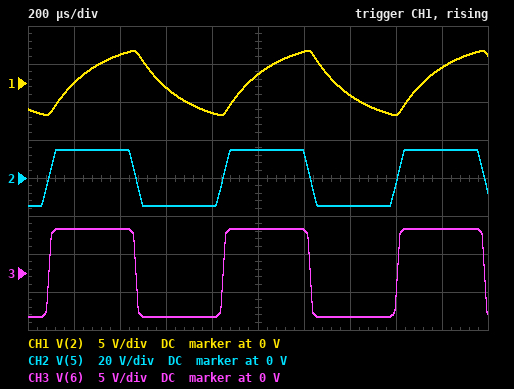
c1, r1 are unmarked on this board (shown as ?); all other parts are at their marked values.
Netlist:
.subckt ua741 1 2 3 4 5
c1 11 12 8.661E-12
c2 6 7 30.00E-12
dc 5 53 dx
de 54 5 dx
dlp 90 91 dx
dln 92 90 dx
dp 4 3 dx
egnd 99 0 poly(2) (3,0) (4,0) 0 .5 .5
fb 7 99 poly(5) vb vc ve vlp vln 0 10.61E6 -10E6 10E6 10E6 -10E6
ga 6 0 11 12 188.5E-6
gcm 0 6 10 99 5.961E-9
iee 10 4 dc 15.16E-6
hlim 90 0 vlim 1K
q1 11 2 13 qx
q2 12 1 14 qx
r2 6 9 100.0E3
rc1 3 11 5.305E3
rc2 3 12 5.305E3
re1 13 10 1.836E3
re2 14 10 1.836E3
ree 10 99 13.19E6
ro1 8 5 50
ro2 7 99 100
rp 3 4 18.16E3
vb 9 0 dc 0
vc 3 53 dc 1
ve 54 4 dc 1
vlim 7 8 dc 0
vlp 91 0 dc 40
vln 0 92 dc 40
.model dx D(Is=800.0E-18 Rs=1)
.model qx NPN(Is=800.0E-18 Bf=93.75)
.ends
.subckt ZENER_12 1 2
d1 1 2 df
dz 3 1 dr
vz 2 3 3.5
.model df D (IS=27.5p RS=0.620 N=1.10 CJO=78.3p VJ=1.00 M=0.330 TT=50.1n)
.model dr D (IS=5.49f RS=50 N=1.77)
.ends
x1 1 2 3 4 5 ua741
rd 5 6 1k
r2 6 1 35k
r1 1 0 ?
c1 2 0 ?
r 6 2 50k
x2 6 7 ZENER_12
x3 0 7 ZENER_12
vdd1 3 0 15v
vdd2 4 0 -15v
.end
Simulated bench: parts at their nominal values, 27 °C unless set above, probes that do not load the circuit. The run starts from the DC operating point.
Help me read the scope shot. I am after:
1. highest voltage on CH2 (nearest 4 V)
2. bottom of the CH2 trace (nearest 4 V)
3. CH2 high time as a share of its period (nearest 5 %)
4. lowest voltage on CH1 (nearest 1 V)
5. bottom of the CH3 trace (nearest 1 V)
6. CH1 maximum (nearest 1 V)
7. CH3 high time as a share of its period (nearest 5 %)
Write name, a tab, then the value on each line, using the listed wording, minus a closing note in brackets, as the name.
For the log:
highest voltage on CH2	16 V
bottom of the CH2 trace	-16 V
CH2 high time as a share of its period	50 %
lowest voltage on CH1	-4 V
bottom of the CH3 trace	-6 V
CH1 maximum	4 V
CH3 high time as a share of its period	50 %
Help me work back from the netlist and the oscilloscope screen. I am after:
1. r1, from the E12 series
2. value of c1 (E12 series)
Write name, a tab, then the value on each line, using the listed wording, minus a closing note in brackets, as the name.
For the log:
r1, from the E12 series	82 kΩ
value of c1	3.9 nF
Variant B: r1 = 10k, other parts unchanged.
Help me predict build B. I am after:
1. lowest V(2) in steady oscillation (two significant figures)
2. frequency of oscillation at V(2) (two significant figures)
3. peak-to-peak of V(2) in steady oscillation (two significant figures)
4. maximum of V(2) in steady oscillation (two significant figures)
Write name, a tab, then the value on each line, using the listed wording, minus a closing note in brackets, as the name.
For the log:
lowest V(2) in steady oscillation	-1.8 V
frequency of oscillation at V(2)	3.6 kHz
peak-to-peak of V(2) in steady oscillation	3.6 V
maximum of V(2) in steady oscillation	1.8 V
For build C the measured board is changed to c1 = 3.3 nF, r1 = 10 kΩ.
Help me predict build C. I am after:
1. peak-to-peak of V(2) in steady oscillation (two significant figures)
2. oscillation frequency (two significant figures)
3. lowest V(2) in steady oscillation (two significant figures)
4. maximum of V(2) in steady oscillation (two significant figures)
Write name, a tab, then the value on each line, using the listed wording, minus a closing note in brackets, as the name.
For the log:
peak-to-peak of V(2) in steady oscillation	3.8 V
oscillation frequency	4.0 kHz
lowest V(2) in steady oscillation	-1.9 V
maximum of V(2) in steady oscillation	1.9 V
